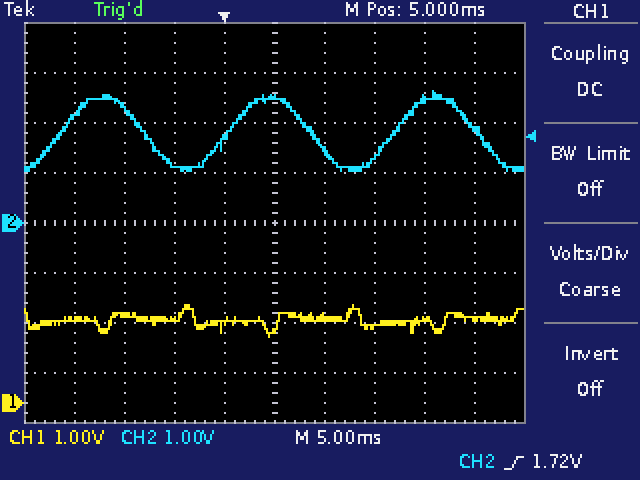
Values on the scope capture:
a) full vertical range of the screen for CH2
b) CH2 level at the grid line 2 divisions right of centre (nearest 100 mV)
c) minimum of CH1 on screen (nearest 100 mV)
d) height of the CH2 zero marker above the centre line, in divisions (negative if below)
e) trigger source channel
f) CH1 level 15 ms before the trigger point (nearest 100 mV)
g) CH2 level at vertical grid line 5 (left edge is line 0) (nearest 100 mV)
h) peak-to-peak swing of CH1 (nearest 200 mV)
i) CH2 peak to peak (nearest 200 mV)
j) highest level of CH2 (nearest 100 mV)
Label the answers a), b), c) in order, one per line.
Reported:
a) 8 V
b) 1.3 V
c) 1.3 V
d) 0.0 div
e) CH2
f) 1.7 V
g) 2.5 V
h) 600 mV
i) 1.6 V
j) 2.6 V
